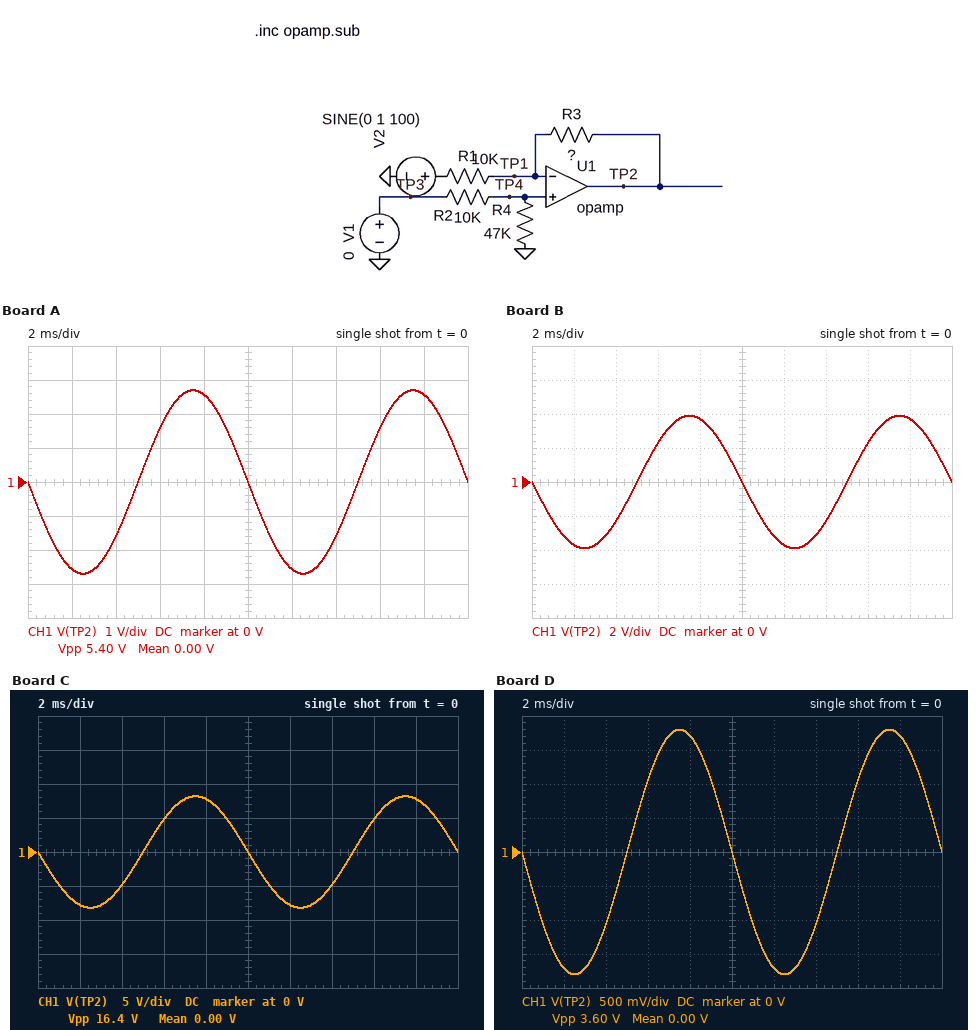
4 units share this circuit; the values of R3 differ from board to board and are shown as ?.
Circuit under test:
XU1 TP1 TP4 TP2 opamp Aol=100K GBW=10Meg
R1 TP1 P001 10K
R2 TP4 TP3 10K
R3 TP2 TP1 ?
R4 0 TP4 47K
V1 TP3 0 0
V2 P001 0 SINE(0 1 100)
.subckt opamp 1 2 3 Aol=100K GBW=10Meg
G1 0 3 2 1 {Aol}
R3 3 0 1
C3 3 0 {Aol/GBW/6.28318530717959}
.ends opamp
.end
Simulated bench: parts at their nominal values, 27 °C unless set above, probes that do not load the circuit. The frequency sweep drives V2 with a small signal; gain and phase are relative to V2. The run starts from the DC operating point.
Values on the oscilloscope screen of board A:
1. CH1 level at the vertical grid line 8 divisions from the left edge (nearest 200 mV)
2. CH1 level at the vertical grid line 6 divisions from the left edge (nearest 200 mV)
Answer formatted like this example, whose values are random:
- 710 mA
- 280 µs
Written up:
- 1.6 V
- -2.6 V
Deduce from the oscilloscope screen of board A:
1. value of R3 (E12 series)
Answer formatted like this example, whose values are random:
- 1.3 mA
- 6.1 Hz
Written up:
- 27 kΩ
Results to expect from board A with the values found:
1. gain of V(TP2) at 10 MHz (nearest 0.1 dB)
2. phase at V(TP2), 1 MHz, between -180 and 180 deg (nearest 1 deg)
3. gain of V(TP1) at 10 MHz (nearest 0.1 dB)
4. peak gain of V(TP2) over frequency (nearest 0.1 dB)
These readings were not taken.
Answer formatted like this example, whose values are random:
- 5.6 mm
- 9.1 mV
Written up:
- -3.0 dB
- 160 deg
- -3.0 dB
- 8.6 dB
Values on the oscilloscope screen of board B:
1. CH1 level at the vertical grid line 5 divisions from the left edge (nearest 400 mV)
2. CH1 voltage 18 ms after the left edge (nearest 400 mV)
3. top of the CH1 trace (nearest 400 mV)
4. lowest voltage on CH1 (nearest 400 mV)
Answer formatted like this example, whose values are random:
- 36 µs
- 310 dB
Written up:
- 0 V
- 3.6 V
- 4.0 V
- -4.0 V
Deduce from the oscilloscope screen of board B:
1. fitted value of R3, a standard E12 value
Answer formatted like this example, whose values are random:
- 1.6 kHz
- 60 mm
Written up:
- 39 kΩ
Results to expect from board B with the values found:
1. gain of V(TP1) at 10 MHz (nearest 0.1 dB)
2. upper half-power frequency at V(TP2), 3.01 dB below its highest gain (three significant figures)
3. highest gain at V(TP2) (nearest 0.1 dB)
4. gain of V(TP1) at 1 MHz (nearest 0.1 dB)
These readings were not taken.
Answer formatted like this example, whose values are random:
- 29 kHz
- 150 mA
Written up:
- -2.2 dB
- 2.04 MHz
- 11.8 dB
- -9.1 dB
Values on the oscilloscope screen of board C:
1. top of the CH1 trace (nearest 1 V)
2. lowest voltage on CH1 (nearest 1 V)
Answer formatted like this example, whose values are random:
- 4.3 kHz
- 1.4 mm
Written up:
- 8 V
- -8 V
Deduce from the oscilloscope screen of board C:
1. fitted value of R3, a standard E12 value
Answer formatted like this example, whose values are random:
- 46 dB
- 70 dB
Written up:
- 82 kΩ
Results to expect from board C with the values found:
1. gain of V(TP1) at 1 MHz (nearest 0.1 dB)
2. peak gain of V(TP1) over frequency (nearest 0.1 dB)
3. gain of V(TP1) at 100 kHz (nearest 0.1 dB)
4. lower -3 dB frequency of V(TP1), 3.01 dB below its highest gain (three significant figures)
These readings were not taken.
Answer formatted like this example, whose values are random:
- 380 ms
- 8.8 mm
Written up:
- -4.4 dB
- -1.0 dB
- -21.8 dB
- 1.09 MHz
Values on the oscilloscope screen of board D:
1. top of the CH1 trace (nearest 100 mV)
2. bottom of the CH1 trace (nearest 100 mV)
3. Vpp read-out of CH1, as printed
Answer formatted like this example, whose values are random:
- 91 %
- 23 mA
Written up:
- 1.8 V
- -1.8 V
- 3.60 V
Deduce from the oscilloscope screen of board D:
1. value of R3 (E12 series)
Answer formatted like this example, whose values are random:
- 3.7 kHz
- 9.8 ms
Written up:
- 18 kΩ
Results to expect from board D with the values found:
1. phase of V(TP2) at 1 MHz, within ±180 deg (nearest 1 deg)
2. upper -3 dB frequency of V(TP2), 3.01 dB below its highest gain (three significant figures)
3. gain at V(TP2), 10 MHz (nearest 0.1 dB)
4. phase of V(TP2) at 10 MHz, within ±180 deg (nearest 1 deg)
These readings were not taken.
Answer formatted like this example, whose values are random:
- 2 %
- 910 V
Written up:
- 164 deg
- 3.57 MHz
- -4.4 dB
- 110 deg
